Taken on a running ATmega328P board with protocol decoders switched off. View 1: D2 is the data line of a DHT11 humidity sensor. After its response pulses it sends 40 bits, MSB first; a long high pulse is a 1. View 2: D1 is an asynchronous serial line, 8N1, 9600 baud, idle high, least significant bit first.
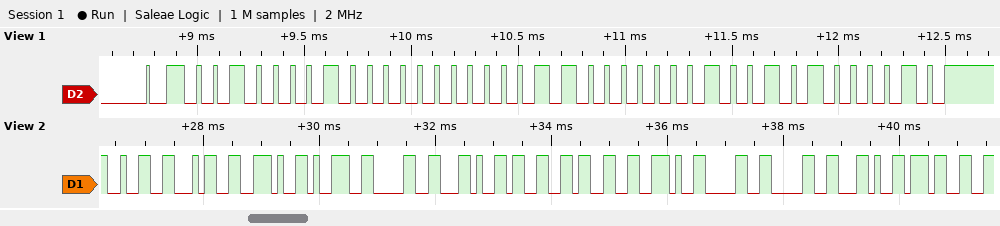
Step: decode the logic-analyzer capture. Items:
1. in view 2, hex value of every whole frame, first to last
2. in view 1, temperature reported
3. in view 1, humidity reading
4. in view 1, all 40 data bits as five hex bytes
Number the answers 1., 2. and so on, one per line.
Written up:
1. 0x32 0x34 0x2E 0x39 0x30 0x2C 0x33 0x33 0x2E 0x30 0x30 0x2C 0x37
2. 24.9 °C
3. 33 %
4. 21 00 18 09 42
